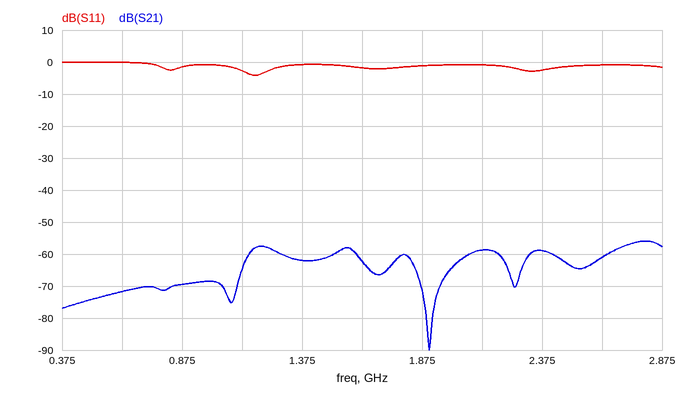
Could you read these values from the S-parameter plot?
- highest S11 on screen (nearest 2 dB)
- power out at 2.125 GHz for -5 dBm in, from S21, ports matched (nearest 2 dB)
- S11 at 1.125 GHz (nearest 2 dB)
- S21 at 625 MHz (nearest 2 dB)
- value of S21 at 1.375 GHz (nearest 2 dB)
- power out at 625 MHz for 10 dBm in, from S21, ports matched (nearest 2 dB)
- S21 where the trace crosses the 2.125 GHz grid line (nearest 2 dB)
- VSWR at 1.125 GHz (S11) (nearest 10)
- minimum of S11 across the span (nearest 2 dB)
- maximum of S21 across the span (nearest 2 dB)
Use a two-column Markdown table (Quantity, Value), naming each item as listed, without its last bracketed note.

| Quantity | Value |
|---|---|
| highest S11 on screen | 0 dB |
| power out at 2.125 GHz for -5 dBm in, from S21, ports matched | -64 dBm |
| S11 at 1.125 GHz | -2 dB |
| S21 at 625 MHz | -72 dB |
| value of S21 at 1.375 GHz | -62 dB |
| power out at 625 MHz for 10 dBm in, from S21, ports matched | -62 dBm |
| S21 where the trace crosses the 2.125 GHz grid line | -58 dB |
| VSWR at 1.125 GHz (S11) | 10 |
| minimum of S11 across the span | -4 dB |
| maximum of S21 across the span | -56 dB |
